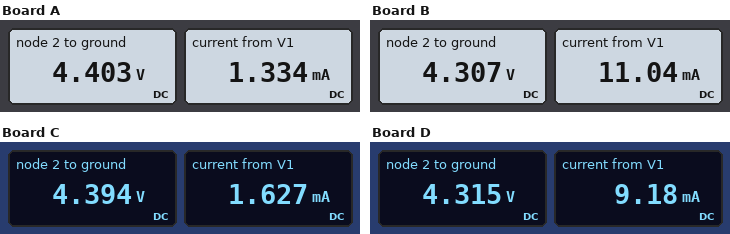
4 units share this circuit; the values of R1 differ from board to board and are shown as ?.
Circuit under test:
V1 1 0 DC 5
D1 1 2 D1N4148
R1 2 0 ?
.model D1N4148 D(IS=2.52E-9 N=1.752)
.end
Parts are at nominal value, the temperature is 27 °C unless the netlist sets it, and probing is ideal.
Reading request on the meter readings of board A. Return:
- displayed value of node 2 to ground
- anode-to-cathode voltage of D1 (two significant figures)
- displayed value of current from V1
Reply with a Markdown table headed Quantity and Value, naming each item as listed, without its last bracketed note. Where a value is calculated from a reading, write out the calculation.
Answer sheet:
| Quantity | Value |
|---|---|
| displayed value of node 2 to ground | 4.403 V |
| anode-to-cathode voltage of D1 | 5 V - 4.403 V = 600 mV |
| displayed value of current from V1 | 1.334 mA |
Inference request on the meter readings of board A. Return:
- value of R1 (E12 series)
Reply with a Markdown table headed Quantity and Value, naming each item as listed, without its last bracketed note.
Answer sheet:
| Quantity | Value |
|---|---|
| value of R1 | 3.3 kΩ |
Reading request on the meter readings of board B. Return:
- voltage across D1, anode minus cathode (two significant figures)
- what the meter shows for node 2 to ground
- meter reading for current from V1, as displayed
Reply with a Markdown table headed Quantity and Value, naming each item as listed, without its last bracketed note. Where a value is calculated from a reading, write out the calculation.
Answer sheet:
| Quantity | Value |
|---|---|
| voltage across D1, anode minus cathode | 5 V - 4.307 V = 690 mV |
| what the meter shows for node 2 to ground | 4.307 V |
| meter reading for current from V1, as displayed | 11.04 mA |
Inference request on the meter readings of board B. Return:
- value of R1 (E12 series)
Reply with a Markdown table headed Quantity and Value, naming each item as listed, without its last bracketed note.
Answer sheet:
| Quantity | Value |
|---|---|
| value of R1 | 390 Ω |
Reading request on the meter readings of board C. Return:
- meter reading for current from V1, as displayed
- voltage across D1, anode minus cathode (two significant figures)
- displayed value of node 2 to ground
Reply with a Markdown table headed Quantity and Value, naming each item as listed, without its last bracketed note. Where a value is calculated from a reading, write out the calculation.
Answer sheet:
| Quantity | Value |
|---|---|
| meter reading for current from V1, as displayed | 1.627 mA |
| voltage across D1, anode minus cathode | 5 V - 4.394 V = 610 mV |
| displayed value of node 2 to ground | 4.394 V |
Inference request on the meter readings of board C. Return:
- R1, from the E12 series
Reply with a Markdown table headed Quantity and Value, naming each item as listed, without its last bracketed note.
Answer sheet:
| Quantity | Value |
|---|---|
| R1, from the E12 series | 2.7 kΩ |
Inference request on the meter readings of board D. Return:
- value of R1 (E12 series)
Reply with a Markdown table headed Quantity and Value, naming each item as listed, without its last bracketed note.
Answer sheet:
| Quantity | Value |
|---|---|
| value of R1 | 470 Ω |
